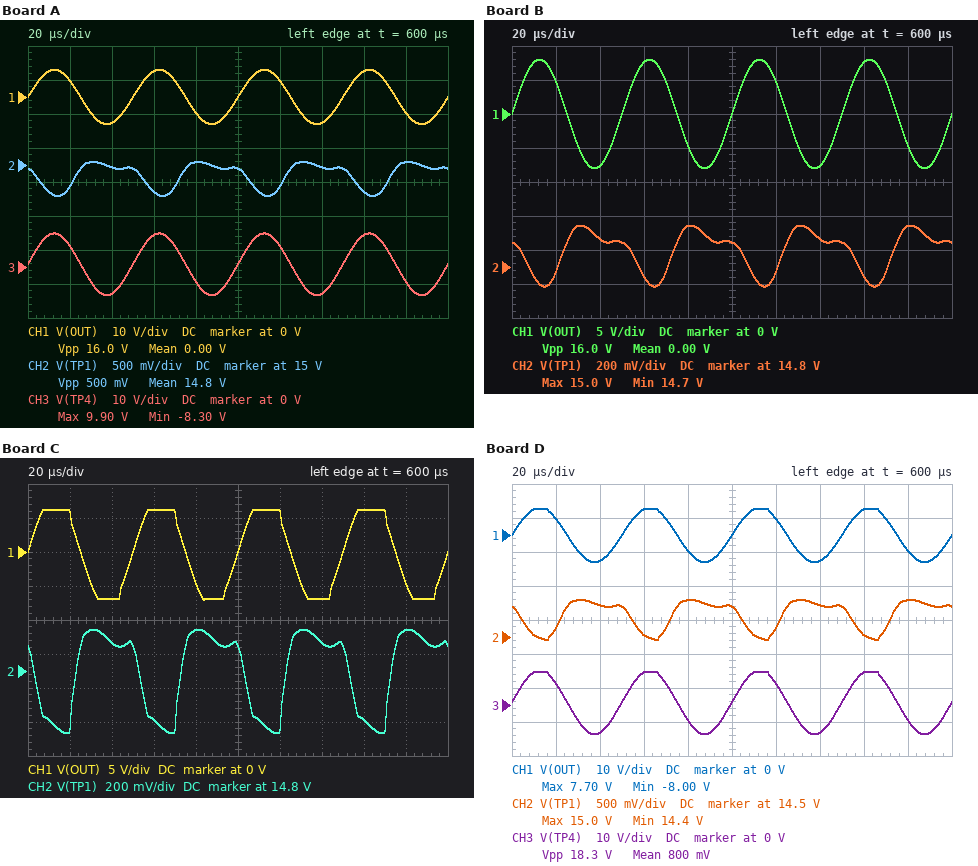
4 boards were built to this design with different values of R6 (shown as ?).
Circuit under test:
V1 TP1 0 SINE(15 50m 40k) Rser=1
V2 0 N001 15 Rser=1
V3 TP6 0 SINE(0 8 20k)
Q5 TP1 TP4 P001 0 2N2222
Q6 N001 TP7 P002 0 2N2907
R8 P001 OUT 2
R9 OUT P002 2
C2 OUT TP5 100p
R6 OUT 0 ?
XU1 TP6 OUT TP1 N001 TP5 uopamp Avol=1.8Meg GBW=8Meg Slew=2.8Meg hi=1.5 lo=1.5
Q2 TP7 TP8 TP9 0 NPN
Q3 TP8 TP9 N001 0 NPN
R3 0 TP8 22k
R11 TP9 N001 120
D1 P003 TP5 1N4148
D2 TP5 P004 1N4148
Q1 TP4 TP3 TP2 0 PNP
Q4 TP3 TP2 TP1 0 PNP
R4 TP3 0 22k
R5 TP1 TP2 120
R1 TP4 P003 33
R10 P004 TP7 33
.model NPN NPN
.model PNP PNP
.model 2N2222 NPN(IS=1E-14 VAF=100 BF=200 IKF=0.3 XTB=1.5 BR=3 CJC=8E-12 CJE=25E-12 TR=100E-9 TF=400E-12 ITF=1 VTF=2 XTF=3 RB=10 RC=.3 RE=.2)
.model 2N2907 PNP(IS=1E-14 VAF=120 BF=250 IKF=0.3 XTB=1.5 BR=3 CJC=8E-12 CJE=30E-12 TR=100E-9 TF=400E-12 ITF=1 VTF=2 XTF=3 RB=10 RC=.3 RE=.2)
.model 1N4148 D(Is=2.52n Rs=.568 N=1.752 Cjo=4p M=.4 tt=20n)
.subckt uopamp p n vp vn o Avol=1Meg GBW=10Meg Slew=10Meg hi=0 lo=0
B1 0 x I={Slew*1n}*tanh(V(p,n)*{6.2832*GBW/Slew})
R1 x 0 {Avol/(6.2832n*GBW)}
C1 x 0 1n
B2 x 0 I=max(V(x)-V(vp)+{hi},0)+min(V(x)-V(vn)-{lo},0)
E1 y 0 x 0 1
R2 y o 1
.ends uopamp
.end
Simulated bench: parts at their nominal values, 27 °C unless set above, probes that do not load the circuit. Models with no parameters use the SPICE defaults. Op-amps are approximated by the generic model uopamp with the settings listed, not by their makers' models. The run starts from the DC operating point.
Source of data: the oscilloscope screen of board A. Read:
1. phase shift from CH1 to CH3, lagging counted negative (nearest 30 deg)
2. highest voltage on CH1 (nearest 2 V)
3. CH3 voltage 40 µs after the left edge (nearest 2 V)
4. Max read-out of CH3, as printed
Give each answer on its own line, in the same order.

0 deg
8 V
-8 V
9.90 V
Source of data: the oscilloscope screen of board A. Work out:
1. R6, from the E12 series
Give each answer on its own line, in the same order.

18 Ω
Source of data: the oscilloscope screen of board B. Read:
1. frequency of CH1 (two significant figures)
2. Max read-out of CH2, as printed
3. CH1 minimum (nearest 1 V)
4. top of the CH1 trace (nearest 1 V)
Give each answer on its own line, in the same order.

20 kHz
15.0 V
-8 V
8 V
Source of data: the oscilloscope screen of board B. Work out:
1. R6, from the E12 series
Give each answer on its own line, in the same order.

27 Ω
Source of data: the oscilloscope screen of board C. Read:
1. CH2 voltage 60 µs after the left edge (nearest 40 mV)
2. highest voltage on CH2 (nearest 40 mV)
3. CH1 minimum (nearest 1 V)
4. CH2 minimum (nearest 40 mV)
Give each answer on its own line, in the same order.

14.52 V
15.04 V
-7 V
14.44 V
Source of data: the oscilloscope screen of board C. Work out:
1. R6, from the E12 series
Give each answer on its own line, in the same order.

12 Ω
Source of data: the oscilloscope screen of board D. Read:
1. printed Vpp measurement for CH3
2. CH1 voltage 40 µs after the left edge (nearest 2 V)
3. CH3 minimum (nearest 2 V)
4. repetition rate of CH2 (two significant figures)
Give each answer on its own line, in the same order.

18.3 V
-8 V
-8 V
20 kHz
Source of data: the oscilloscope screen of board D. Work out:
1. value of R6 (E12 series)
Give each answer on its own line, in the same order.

15 Ω
